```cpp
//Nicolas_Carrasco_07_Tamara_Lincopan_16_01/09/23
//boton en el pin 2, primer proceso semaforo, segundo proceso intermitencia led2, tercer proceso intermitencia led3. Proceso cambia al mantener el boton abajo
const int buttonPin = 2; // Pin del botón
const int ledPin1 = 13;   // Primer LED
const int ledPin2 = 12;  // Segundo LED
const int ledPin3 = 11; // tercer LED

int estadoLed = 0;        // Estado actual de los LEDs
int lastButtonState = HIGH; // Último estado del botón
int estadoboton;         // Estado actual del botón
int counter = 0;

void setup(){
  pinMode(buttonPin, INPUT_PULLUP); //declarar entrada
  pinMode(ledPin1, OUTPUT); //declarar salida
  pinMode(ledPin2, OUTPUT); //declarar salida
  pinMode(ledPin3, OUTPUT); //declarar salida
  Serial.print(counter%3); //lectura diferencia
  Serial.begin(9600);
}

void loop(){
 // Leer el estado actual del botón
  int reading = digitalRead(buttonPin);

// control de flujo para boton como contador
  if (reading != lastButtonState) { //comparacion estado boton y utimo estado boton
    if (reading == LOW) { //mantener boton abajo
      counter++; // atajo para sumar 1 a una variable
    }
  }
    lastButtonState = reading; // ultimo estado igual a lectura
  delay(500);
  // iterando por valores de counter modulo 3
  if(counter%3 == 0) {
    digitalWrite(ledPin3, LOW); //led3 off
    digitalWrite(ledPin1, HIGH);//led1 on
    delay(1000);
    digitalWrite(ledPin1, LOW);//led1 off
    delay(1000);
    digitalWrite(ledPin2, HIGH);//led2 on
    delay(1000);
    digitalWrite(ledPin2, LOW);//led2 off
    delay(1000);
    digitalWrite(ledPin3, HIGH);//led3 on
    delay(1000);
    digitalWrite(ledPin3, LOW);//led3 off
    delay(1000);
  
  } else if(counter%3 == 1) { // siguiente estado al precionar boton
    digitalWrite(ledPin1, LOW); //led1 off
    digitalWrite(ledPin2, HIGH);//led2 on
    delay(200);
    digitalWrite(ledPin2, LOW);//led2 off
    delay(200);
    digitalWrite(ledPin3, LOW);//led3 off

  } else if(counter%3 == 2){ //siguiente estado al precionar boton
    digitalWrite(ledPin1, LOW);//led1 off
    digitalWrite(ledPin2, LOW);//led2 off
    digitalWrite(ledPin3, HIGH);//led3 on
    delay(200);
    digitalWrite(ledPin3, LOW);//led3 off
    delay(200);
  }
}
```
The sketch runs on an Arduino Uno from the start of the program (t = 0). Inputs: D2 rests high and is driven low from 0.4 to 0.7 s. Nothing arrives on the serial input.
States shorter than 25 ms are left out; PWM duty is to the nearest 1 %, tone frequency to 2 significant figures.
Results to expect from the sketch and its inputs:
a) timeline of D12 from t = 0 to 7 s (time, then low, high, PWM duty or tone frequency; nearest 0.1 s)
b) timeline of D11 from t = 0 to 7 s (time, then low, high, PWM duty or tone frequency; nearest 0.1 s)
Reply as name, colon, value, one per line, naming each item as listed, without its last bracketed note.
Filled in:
timeline of D12 from t = 0 to 7 s: 0 s low; 2.5 s high; 3.5 s low
timeline of D11 from t = 0 to 7 s: 0 s low; 4.5 s high; 5.5 s low
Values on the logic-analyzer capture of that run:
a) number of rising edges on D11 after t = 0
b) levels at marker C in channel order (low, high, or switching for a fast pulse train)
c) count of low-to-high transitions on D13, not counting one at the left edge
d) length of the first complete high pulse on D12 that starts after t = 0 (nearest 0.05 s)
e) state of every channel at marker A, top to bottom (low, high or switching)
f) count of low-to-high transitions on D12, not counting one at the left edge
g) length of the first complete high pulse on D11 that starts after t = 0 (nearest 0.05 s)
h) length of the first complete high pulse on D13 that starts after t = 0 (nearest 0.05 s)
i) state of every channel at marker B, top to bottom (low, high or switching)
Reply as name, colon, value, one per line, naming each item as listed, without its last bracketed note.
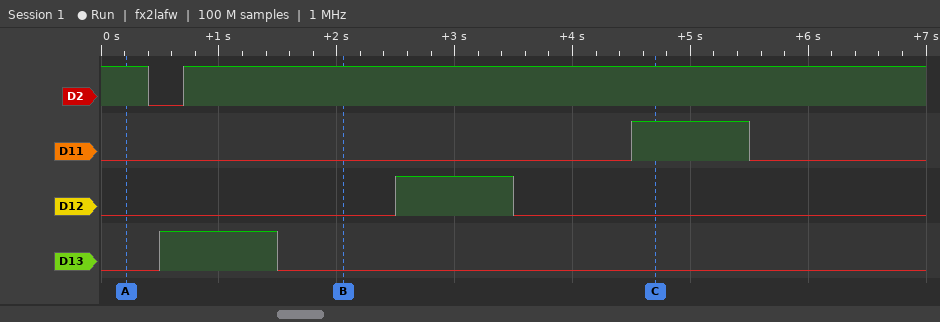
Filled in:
number of rising edges on D11 after t = 0: 1
levels at marker C in channel order: D2 high, D11 high, D12 low, D13 low
count of low-to-high transitions on D13, not counting one at the left edge: 1
length of the first complete high pulse on D12 that starts after t = 0: 1.00 s
state of every channel at marker A, top to bottom: D2 high, D11 low, D12 low, D13 low
count of low-to-high transitions on D12, not counting one at the left edge: 1
length of the first complete high pulse on D11 that starts after t = 0: 1.00 s
length of the first complete high pulse on D13 that starts after t = 0: 1.00 s
state of every channel at marker B, top to bottom: D2 high, D11 low, D12 low, D13 low
